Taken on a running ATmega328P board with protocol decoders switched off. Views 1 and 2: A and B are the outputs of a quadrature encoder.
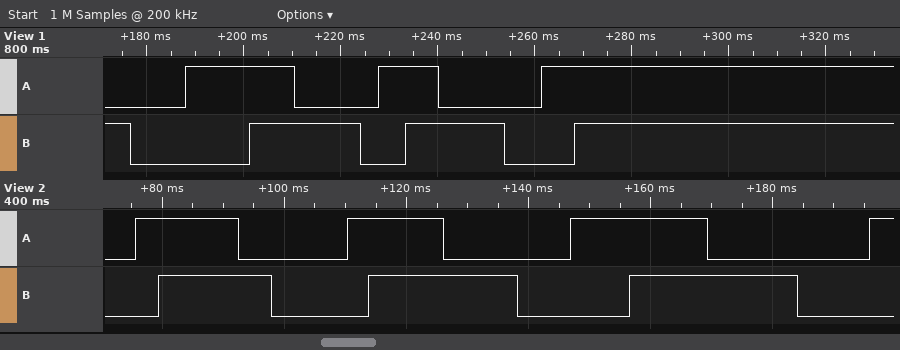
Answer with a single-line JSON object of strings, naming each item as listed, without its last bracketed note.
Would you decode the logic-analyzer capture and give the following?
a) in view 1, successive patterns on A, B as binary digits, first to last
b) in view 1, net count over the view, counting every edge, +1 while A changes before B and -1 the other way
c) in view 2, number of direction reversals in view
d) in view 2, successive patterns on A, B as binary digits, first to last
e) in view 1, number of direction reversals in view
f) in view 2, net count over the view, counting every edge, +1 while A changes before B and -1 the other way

{"in view 1, successive patterns on A, B as binary digits, first to last": "01 00 10 11 01 00 10 11 01 00 10 11", "in view 1, net count over the view, counting every edge, +1 while A changes before B and -1 the other way": "+11", "in view 2, number of direction reversals in view": "0", "in view 2, successive patterns on A, B as binary digits, first to last": "00 10 11 01 00 10 11 01 00 10 11 01 00 10", "in view 1, number of direction reversals in view": "0", "in view 2, net count over the view, counting every edge, +1 while A changes before B and -1 the other way": "+13"}
